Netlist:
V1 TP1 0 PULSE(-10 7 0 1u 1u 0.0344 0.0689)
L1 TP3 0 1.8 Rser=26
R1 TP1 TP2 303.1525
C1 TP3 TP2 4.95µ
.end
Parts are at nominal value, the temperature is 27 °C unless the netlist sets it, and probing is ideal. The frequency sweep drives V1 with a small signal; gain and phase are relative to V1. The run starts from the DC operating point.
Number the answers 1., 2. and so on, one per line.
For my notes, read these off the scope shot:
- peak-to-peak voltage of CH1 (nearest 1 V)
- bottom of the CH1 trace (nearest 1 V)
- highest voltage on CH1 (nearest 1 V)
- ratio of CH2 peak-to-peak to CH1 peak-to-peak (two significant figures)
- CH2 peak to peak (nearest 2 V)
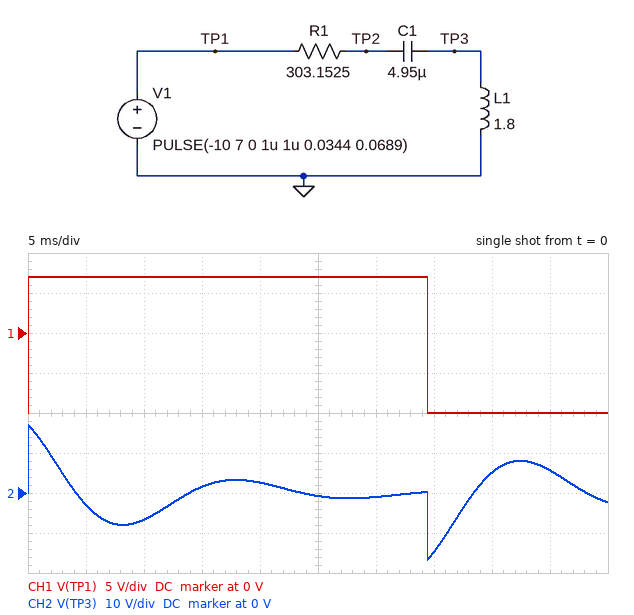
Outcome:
1. 17 V
2. -10 V
3. 7 V
4. 2.0
5. 34 V
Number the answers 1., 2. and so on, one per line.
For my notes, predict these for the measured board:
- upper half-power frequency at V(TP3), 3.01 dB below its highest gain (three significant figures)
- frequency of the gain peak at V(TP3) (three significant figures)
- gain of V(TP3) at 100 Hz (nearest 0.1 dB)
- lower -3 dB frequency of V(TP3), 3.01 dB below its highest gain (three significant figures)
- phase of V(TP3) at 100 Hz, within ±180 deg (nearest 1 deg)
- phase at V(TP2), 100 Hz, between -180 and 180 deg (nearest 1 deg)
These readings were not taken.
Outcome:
1. 93.3 Hz
2. 57.8 Hz
3. 2.2 dB
4. 45.4 Hz
5. 21 deg
6. 20 deg
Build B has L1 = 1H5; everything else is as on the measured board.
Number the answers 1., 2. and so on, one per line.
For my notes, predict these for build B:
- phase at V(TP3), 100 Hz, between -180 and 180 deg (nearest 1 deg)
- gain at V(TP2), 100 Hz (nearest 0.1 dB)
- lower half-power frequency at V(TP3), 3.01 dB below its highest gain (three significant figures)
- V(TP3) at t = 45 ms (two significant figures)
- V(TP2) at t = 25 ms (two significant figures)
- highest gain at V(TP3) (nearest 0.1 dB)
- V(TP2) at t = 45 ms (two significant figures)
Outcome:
1. 26 deg
2. -1.1 dB
3. 49.5 Hz
4. 3.6 V
5. 6.6 V
6. 4.9 dB
7. -12 V
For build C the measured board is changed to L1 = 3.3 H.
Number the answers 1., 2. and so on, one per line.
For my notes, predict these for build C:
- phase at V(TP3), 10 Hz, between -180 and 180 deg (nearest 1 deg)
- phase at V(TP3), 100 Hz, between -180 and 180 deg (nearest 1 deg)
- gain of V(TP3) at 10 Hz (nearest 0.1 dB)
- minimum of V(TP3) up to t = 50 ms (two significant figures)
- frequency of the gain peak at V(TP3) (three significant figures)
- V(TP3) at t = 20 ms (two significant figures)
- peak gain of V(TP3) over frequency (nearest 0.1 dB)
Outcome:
1. 167 deg
2. 10 deg
3. -23.2 dB
4. -19 V
5. 41.1 Hz
6. 1.9 V
7. 8.1 dB
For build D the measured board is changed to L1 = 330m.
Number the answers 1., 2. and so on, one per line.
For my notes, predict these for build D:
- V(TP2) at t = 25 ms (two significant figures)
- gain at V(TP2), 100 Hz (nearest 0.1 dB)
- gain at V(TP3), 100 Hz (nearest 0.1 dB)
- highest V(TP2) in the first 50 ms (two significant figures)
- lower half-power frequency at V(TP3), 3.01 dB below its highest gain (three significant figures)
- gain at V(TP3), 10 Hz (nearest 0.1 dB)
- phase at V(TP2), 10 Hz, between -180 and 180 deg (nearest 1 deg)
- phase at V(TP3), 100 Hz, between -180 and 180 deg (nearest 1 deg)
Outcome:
1. 7.0 V
2. -9.5 dB
3. -4.4 dB
4. 7.7 V
5. 115 Hz
6. -39.7 dB
7. -5 deg
8. 102 deg
